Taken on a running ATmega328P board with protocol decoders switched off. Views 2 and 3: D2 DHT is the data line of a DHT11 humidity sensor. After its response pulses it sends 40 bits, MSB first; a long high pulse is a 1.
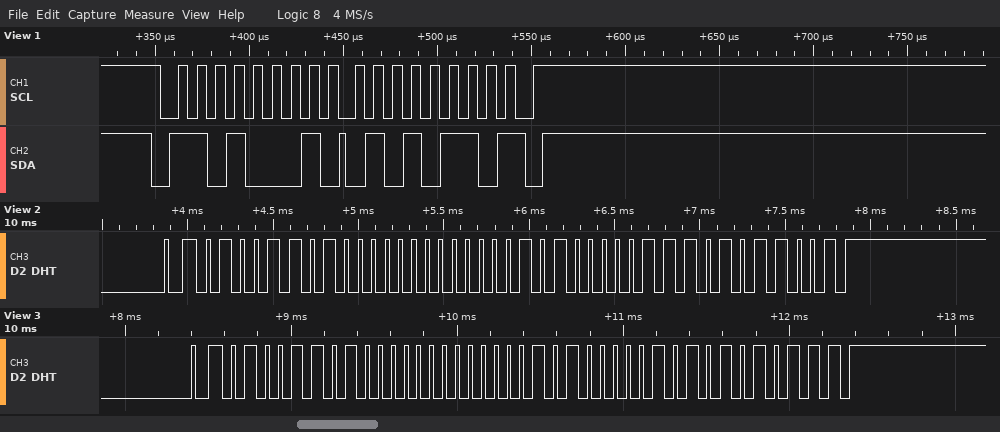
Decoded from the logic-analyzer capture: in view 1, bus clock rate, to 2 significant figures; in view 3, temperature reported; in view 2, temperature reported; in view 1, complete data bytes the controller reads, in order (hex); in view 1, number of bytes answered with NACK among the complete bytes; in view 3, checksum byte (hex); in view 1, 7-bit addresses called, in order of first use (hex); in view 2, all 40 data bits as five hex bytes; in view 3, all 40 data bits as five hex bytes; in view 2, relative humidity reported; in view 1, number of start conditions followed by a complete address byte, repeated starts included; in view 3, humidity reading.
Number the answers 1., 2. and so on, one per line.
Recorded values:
1. 100 kHz
2. 5.5 °C
3. 5.7 °C
4. 56
5. 1
6. 0x57
7. 0x68
8. 4D 00 05 07 59
9. 4D 00 05 05 57
10. 77 %
11. 1
12. 77 %
